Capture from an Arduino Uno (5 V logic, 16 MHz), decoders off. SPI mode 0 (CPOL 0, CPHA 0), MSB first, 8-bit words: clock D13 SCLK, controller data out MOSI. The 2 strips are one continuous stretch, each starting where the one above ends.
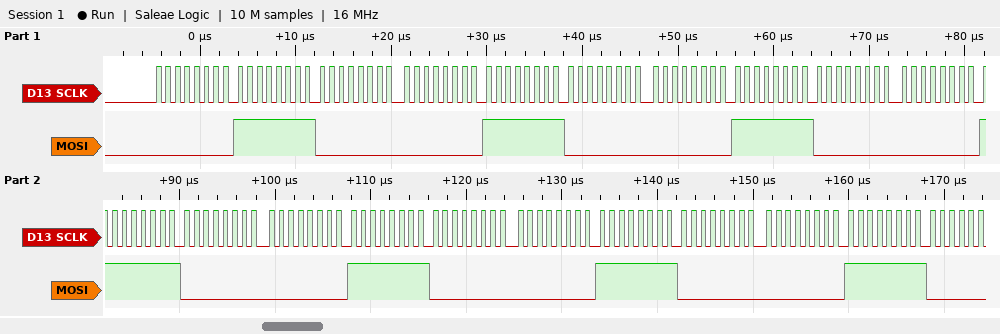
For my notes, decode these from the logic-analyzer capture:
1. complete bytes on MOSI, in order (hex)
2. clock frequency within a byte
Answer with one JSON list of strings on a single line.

["00 FF 00 00 FF 00 00 FF 00 00 FF 00 00 FF 00 00 FF 00 00 FF", "1 MHz"]
